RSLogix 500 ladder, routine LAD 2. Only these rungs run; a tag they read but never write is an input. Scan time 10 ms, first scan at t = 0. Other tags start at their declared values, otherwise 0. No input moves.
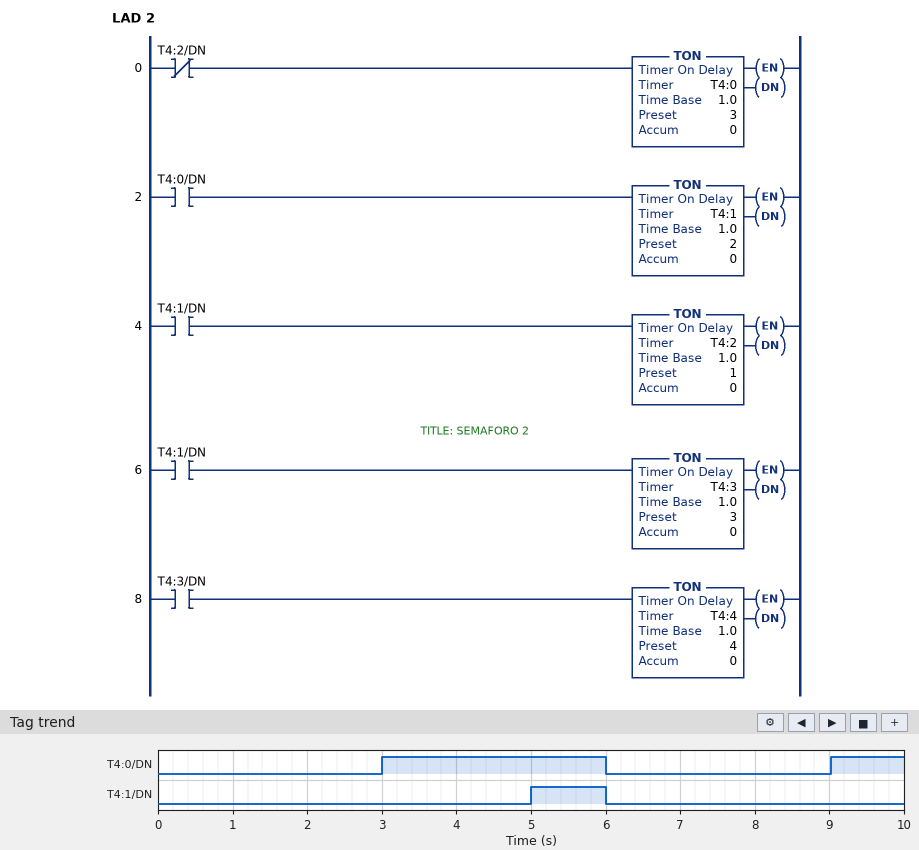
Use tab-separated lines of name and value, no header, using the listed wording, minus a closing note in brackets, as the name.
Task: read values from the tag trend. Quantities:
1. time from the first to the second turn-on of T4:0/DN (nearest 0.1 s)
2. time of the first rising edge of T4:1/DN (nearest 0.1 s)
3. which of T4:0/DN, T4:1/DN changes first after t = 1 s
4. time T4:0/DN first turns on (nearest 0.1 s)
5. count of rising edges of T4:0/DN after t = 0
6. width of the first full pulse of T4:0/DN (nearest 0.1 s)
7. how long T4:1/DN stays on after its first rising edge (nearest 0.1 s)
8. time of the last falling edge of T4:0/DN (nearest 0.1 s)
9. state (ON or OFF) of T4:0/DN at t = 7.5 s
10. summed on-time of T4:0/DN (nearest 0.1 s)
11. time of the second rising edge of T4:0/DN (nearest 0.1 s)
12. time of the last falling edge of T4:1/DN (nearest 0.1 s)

time from the first to the second turn-on of T4:0/DN	6.0 s
time of the first rising edge of T4:1/DN	5.0 s
which of T4:0/DN, T4:1/DN changes first after t = 1 s	T4:0/DN
time T4:0/DN first turns on	3.0 s
count of rising edges of T4:0/DN after t = 0	2
width of the first full pulse of T4:0/DN	3.0 s
how long T4:1/DN stays on after its first rising edge	1.0 s
time of the last falling edge of T4:0/DN	6.0 s
state (ON or OFF) of T4:0/DN at t = 7.5 s	OFF
summed on-time of T4:0/DN	4.0 s
time of the second rising edge of T4:0/DN	9.0 s
time of the last falling edge of T4:1/DN	6.0 s
